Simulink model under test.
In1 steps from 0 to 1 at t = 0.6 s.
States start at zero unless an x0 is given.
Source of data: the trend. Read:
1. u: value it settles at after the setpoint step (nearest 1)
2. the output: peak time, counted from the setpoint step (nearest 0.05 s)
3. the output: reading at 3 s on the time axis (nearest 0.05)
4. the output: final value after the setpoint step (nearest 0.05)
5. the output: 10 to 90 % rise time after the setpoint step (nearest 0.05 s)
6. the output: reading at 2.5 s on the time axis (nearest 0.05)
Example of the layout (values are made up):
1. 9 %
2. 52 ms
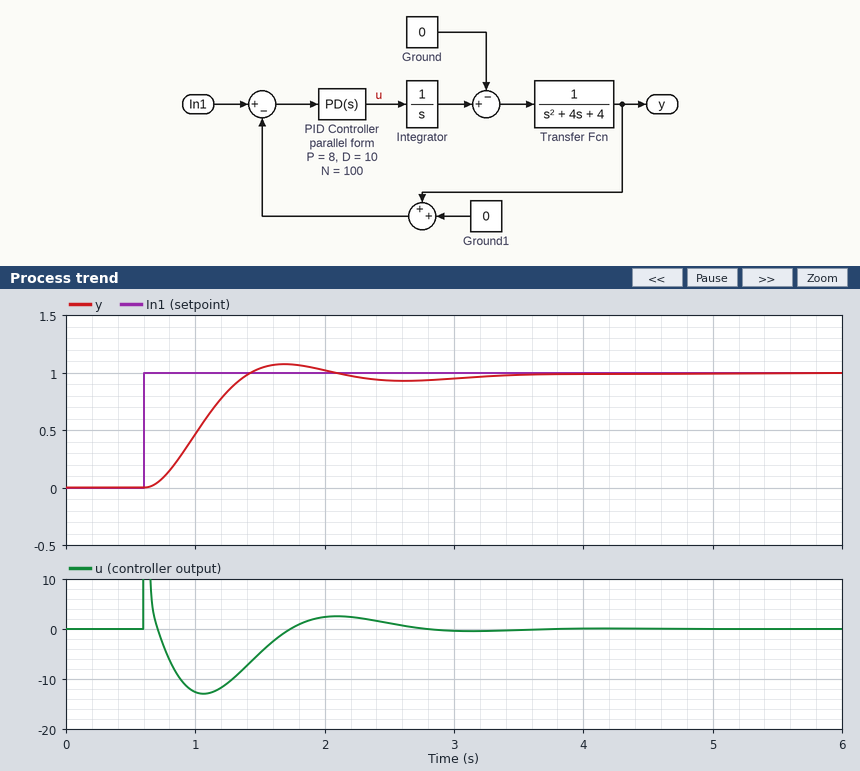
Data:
1. 0
2. 1.10 s
3. 0.95
4. 1.00
5. 0.55 s
6. 0.95
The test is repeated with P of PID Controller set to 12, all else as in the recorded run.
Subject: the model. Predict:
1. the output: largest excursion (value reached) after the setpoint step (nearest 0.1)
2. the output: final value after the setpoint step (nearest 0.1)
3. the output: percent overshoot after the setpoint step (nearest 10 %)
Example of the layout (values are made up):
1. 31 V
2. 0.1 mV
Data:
1. 1.2
2. 1.0
3. 20 %
